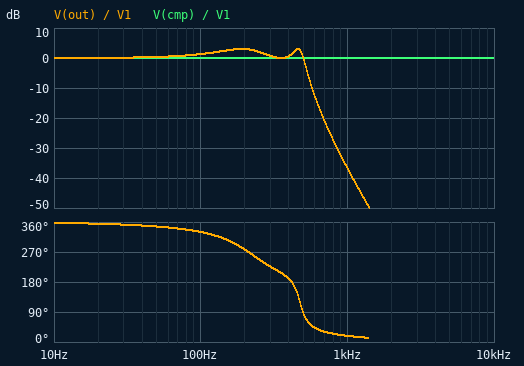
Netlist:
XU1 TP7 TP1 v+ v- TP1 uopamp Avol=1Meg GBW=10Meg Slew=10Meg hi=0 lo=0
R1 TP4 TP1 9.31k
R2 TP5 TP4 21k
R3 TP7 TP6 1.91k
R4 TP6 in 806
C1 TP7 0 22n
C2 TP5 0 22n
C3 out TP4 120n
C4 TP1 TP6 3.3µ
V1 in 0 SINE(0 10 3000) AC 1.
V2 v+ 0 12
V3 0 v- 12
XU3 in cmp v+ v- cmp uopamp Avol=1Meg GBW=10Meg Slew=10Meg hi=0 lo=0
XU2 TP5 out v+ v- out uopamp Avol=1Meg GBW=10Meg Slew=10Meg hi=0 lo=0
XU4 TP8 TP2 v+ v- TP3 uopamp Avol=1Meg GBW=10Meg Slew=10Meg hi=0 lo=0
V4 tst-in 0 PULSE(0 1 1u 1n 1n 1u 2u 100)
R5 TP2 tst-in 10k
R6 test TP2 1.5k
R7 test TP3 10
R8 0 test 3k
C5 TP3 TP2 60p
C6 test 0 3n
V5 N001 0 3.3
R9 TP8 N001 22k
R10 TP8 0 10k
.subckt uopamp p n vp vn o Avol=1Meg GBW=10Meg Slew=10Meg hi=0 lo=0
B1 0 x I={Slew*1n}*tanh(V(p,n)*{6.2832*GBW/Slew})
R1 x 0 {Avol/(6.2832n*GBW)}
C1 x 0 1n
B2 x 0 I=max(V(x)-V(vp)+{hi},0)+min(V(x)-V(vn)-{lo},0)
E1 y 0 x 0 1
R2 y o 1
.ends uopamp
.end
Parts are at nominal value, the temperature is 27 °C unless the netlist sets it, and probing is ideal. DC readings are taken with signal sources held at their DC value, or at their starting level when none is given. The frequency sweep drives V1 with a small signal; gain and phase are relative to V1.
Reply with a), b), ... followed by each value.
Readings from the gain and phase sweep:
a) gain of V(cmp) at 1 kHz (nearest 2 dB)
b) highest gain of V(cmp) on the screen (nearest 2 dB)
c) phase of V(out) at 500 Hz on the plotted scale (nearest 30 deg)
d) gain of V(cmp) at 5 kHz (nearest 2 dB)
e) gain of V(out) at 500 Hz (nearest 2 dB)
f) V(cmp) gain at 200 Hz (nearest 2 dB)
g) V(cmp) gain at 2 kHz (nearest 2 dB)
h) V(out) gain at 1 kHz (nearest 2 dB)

a) 0 dB
b) 0 dB
c) 90 deg
d) 0 dB
e) 0 dB
f) 0 dB
g) 0 dB
h) -36 dB
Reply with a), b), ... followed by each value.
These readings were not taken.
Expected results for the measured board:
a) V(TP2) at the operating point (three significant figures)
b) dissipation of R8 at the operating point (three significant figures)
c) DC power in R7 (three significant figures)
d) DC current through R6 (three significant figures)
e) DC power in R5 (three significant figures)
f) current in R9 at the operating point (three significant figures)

a) 1.03 V
b) 469 µW
c) 2.48 µW
d) 103 µA
e) 106 µW
f) 103 µA
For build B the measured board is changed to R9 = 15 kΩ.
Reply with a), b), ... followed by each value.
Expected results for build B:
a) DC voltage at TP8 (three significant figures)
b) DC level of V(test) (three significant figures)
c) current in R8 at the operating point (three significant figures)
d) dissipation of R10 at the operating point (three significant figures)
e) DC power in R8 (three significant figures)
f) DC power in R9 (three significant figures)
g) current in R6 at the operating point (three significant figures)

a) 1.32 V
b) 1.52 V
c) 506 µA
d) 174 µW
e) 768 µW
f) 261 µW
g) 132 µA
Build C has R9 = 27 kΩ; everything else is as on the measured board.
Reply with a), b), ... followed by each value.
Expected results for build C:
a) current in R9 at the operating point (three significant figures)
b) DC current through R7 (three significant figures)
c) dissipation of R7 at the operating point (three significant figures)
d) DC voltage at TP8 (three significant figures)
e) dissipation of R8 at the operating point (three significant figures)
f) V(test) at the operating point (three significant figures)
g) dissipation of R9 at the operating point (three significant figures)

a) 89.2 µA
b) 431 µA
c) 1.86 µW
d) 892 mV
e) 351 µW
f) 1.03 V
g) 215 µW
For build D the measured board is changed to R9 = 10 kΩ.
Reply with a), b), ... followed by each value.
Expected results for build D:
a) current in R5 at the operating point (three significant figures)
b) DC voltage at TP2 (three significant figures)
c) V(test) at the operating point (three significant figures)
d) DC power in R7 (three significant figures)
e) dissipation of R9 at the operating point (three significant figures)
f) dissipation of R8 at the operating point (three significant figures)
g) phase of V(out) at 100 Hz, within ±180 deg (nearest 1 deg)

a) 165 µA
b) 1.65 V
c) 1.90 V
d) 6.36 µW
e) 272 µW
f) 1.20 mW
g) -30 deg
